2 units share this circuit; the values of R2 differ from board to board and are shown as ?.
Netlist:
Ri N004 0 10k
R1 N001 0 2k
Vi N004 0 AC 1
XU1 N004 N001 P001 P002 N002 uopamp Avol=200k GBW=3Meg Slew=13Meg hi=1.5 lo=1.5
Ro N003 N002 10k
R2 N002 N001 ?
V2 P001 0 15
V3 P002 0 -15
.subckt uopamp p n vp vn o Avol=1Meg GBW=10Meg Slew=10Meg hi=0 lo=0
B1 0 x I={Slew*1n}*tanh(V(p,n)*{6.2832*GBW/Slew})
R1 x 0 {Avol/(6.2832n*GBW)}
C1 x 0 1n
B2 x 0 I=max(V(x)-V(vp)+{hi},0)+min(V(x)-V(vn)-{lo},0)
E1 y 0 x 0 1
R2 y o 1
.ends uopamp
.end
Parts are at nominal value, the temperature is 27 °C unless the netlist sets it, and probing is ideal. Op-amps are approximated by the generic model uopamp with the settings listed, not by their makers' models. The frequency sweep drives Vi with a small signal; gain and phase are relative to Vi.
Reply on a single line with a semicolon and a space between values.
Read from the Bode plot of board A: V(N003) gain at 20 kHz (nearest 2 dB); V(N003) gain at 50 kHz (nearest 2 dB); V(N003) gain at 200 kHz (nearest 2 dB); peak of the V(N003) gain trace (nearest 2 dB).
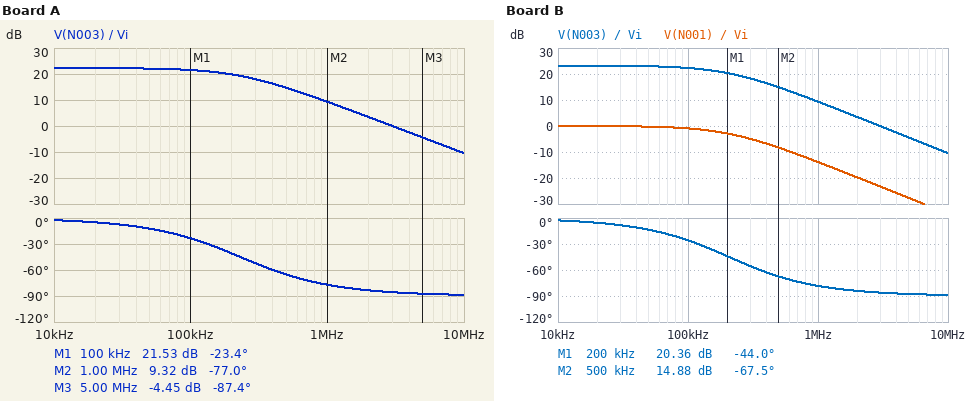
22 dB; 22 dB; 20 dB; 22 dB
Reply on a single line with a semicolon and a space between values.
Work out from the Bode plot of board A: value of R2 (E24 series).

24 kΩ
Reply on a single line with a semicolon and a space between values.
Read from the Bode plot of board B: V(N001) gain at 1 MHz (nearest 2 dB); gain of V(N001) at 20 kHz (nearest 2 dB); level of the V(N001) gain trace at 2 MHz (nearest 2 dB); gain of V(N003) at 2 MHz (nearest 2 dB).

-14 dB; 0 dB; -20 dB; 4 dB
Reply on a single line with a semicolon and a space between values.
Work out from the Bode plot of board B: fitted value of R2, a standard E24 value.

27 kΩ
